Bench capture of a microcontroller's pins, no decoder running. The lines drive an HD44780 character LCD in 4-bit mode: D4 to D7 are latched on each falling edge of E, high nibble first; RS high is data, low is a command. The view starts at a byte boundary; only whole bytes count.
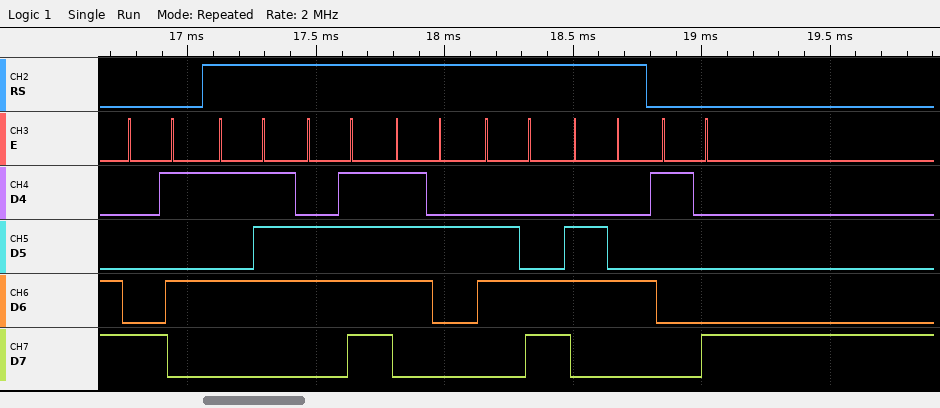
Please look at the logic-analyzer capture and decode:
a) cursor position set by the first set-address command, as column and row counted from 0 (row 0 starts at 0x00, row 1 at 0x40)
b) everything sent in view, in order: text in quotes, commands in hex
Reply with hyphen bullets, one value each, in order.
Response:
- column 5, row 0
- 0x85 "World" 0x18
